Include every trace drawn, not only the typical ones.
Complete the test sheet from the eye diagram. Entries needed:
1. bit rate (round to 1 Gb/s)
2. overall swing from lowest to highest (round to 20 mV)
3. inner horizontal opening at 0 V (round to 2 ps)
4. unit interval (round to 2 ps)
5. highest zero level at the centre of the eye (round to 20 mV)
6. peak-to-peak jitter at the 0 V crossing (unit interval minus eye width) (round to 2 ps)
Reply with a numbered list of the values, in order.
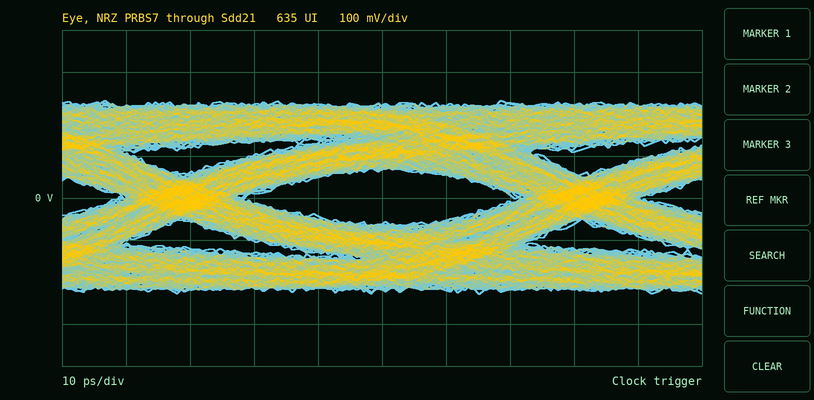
1. 16 Gb/s
2. 460 mV
3. 42 ps
4. 62 ps
5. -60 mV
6. 20 ps
